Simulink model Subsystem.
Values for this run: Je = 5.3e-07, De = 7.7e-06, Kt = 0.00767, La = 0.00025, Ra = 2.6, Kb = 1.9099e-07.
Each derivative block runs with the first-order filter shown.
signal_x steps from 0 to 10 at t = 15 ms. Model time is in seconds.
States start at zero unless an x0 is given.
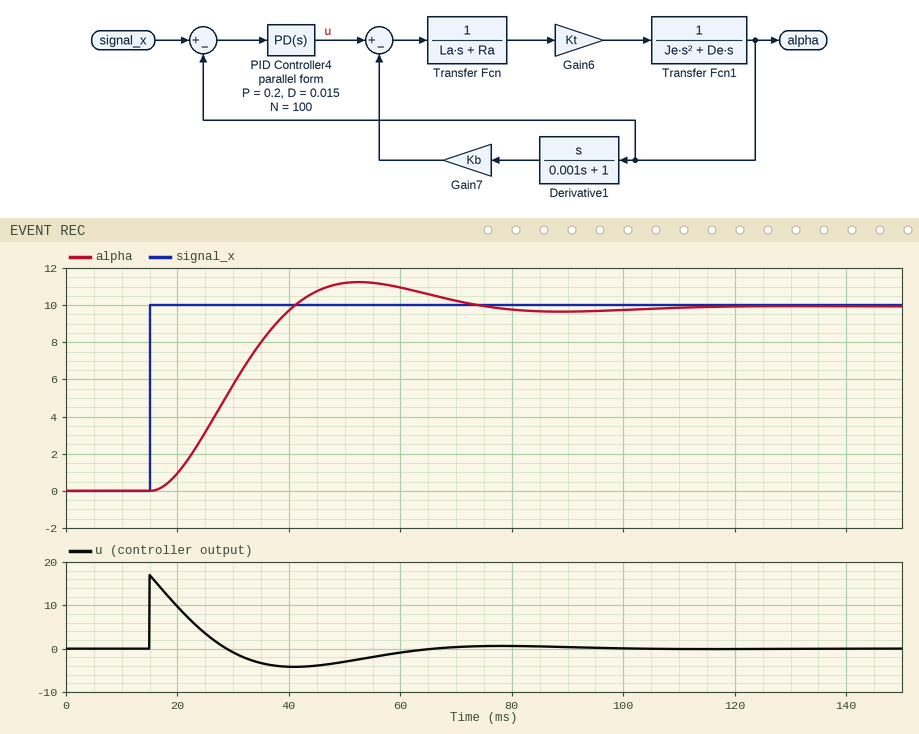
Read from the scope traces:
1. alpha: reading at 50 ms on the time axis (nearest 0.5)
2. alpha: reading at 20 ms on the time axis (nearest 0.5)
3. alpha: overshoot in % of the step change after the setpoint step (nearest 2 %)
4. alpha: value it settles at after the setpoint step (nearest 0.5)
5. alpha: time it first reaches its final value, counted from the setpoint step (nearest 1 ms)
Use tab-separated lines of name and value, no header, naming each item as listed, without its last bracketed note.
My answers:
alpha: reading at 50 ms on the time axis	11.0
alpha: reading at 20 ms on the time axis	1.0
alpha: overshoot in % of the step change after the setpoint step	12 %
alpha: value it settles at after the setpoint step	10.0
alpha: time it first reaches its final value, counted from the setpoint step	26 ms
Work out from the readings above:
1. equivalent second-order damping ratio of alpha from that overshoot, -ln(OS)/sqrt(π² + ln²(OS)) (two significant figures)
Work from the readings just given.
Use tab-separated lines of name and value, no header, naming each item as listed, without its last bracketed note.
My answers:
equivalent second-order damping ratio of alpha from that overshoot, -ln(OS)/sqrt(π² + ln²(OS))	0.56
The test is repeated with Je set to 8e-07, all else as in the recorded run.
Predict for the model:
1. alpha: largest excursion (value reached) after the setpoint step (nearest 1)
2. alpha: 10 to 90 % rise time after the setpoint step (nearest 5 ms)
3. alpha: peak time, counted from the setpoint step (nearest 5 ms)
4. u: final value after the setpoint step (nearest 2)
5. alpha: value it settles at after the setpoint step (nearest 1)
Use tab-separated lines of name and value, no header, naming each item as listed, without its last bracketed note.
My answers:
alpha: largest excursion (value reached) after the setpoint step	11
alpha: 10 to 90 % rise time after the setpoint step	25 ms
alpha: peak time, counted from the setpoint step	50 ms
u: final value after the setpoint step	0
alpha: value it settles at after the setpoint step	10
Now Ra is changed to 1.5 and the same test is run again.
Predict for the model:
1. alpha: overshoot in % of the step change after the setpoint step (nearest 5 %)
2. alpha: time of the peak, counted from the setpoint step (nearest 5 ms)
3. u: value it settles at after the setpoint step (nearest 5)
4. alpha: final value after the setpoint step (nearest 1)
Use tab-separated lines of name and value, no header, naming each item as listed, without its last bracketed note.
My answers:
alpha: overshoot in % of the step change after the setpoint step	25 %
alpha: time of the peak, counted from the setpoint step	25 ms
u: value it settles at after the setpoint step	0
alpha: final value after the setpoint step	10
